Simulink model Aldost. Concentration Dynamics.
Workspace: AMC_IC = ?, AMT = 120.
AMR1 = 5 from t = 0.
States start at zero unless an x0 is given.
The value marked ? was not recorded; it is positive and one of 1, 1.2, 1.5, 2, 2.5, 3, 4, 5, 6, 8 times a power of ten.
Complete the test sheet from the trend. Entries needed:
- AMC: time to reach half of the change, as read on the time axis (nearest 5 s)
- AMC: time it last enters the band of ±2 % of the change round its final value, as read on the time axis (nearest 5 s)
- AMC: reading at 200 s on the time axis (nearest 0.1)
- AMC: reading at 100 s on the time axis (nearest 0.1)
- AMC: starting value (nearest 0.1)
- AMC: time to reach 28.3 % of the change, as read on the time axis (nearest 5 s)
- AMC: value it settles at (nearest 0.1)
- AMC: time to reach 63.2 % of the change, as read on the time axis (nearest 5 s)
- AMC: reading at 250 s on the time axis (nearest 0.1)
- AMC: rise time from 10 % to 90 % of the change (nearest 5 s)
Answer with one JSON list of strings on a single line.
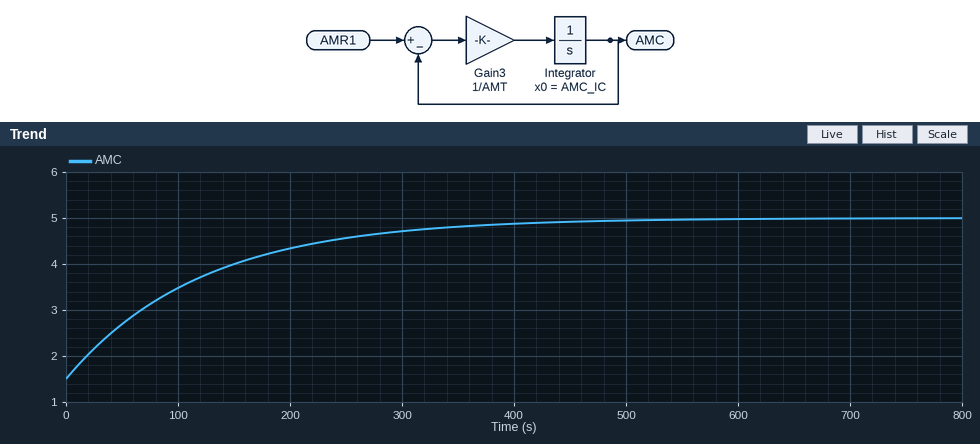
["85 s", "470 s", "4.3", "3.5", "1.5", "40 s", "5.0", "120 s", "4.6", "265 s"]
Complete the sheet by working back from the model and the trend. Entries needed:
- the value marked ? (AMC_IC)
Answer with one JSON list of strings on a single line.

["1.5"]
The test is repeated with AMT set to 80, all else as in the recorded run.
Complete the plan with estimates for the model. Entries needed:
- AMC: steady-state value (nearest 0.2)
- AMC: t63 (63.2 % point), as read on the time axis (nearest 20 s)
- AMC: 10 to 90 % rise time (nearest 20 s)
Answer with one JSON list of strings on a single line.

["5.0", "80 s", "180 s"]
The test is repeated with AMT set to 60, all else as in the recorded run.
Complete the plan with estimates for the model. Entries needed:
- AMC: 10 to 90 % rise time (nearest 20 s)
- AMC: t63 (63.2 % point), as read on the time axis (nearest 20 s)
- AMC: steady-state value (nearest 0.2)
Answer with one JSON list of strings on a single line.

["140 s", "60 s", "5.0"]
